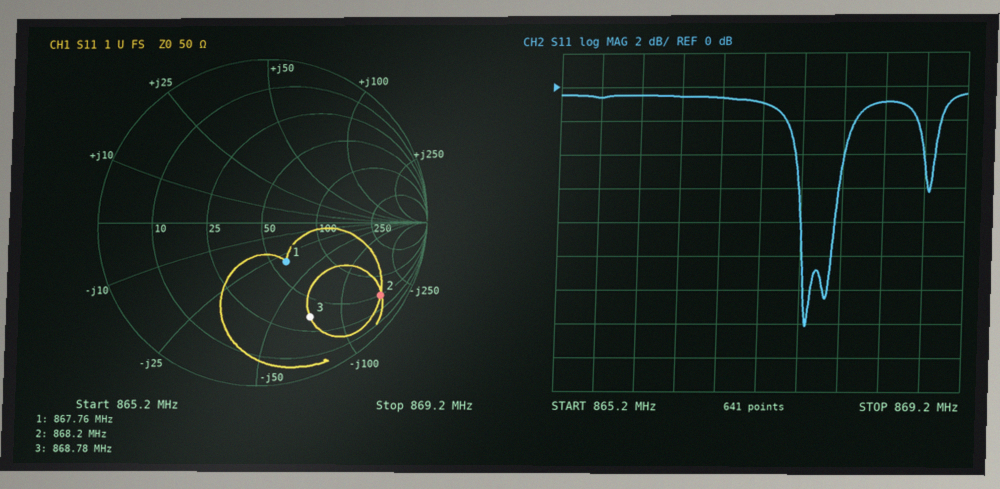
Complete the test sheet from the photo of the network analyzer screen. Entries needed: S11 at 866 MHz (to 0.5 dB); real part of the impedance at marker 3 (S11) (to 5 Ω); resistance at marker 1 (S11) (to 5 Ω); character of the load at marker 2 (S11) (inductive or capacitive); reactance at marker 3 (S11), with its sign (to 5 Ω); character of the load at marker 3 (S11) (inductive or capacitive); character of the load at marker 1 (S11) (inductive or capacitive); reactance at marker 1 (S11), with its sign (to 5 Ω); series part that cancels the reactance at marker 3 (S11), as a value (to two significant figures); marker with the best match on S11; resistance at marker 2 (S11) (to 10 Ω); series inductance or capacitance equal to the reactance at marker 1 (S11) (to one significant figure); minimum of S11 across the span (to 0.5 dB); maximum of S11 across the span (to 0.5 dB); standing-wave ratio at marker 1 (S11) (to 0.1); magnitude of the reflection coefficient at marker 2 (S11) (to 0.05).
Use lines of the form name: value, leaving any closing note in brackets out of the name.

S11 at 866 MHz: -0.5 dB
real part of the impedance at marker 3 (S11): 35 Ω
resistance at marker 1 (S11): 60 Ω
character of the load at marker 2 (S11): capacitive
reactance at marker 3 (S11), with its sign: -70 Ω
character of the load at marker 3 (S11): capacitive
character of the load at marker 1 (S11): capacitive
reactance at marker 1 (S11), with its sign: -30 Ω
series part that cancels the reactance at marker 3 (S11), as a value: 13 nH
marker with the best match on S11: marker 1
resistance at marker 2 (S11): 50 Ω
series inductance or capacitance equal to the reactance at marker 1 (S11): 6 pF
minimum of S11 across the span: -14.0 dB
maximum of S11 across the span: -0.5 dB
standing-wave ratio at marker 1 (S11): 1.8
magnitude of the reflection coefficient at marker 2 (S11): 0.85
